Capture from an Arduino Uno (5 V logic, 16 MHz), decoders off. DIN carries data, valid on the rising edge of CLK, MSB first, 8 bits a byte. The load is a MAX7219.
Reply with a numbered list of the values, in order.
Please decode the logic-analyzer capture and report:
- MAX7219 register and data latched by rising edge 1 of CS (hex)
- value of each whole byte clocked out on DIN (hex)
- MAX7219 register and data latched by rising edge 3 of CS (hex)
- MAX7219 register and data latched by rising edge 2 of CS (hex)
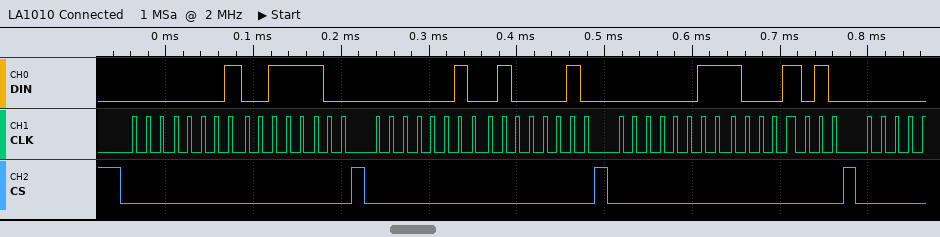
1. register 0x1, data 0x3C
2. 0x01 0x3C 0x02 0x42 0x03 0x8A
3. register 0x3, data 0x8A
4. register 0x2, data 0x42
